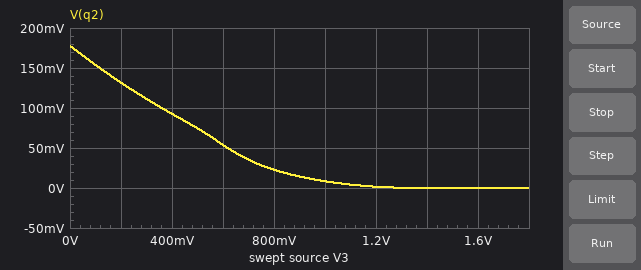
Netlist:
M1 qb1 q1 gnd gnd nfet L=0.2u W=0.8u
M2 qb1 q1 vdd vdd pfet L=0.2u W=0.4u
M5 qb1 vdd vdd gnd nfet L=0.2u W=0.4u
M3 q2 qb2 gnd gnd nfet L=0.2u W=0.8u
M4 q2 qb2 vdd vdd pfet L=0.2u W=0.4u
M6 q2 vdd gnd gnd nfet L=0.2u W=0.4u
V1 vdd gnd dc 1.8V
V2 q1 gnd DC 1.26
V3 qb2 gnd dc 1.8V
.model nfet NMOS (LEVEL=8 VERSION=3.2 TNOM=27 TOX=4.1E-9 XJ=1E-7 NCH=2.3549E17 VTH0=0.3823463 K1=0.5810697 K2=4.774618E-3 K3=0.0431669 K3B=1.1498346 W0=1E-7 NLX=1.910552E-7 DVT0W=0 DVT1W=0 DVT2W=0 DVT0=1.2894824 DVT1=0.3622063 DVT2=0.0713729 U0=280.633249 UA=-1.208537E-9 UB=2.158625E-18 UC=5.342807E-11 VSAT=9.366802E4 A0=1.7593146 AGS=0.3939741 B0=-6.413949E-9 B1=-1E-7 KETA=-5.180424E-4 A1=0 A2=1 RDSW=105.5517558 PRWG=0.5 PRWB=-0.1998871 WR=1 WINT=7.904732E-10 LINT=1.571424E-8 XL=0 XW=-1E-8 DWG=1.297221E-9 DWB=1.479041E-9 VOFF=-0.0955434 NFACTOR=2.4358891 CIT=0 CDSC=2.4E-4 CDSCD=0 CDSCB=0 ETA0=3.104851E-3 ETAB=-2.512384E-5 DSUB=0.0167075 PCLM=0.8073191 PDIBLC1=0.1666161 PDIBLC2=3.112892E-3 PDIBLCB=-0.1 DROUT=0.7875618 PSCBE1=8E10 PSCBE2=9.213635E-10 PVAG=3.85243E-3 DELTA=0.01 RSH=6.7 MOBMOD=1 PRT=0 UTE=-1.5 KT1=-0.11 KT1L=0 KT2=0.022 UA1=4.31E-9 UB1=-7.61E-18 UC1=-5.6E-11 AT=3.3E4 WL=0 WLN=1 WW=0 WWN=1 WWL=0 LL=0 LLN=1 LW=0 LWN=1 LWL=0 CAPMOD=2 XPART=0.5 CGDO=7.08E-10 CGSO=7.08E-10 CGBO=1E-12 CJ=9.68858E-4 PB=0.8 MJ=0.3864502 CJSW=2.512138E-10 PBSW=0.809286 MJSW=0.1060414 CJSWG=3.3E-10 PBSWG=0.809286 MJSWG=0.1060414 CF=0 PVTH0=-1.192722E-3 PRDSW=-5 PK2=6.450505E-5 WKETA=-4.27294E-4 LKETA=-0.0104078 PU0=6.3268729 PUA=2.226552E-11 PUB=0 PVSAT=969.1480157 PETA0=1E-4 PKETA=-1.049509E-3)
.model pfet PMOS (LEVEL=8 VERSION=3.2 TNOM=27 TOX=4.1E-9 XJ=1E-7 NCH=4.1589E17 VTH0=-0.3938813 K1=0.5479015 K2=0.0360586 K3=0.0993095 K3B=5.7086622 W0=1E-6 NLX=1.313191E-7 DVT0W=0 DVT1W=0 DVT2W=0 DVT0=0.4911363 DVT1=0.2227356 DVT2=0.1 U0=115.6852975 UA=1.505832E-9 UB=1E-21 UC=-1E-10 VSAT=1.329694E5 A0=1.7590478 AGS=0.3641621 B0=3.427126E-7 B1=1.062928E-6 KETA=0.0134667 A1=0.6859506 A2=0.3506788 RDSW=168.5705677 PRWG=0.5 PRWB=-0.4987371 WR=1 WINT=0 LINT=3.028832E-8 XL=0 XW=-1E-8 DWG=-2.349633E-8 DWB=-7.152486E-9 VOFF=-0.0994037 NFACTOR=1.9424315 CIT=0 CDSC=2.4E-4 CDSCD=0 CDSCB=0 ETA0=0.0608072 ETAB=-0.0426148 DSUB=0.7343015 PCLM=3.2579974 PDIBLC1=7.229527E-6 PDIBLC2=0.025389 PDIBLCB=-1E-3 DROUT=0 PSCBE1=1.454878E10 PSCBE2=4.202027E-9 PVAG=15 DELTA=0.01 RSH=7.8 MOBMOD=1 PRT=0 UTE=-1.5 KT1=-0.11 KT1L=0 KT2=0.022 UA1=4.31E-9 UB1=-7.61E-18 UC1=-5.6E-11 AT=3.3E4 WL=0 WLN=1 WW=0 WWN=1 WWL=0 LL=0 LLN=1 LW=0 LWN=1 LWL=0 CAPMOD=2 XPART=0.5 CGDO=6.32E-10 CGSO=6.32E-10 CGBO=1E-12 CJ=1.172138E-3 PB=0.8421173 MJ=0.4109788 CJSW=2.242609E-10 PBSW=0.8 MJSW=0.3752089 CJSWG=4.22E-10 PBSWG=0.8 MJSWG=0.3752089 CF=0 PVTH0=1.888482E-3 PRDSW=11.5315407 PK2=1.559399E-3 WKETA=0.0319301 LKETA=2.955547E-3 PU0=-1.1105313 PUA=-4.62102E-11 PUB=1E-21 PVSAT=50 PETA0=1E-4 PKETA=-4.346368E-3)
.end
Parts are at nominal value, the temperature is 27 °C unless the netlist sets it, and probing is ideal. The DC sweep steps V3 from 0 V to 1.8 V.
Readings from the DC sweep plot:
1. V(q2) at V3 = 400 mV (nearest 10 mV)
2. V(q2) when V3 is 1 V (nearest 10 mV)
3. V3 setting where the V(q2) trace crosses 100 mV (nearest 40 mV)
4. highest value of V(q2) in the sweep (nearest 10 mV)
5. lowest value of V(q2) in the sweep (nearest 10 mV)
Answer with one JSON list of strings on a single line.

["90 mV", "10 mV", "360 mV", "180 mV", "0 V"]
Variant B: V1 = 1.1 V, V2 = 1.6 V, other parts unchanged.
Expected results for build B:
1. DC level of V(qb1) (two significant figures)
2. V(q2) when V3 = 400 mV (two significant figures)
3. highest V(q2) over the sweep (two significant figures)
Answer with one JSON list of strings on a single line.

["61 mV", "13 mV", "83 mV"]
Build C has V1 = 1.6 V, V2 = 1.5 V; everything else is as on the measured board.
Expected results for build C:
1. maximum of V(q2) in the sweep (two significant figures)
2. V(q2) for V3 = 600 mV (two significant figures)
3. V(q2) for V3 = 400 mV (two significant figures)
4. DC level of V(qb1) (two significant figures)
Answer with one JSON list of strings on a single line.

["150 mV", "33 mV", "67 mV", "160 mV"]
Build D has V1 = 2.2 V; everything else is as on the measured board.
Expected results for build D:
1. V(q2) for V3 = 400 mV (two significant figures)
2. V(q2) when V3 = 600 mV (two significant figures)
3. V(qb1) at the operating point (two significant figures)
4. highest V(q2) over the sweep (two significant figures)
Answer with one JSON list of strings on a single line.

["150 mV", "110 mV", "510 mV", "250 mV"]
